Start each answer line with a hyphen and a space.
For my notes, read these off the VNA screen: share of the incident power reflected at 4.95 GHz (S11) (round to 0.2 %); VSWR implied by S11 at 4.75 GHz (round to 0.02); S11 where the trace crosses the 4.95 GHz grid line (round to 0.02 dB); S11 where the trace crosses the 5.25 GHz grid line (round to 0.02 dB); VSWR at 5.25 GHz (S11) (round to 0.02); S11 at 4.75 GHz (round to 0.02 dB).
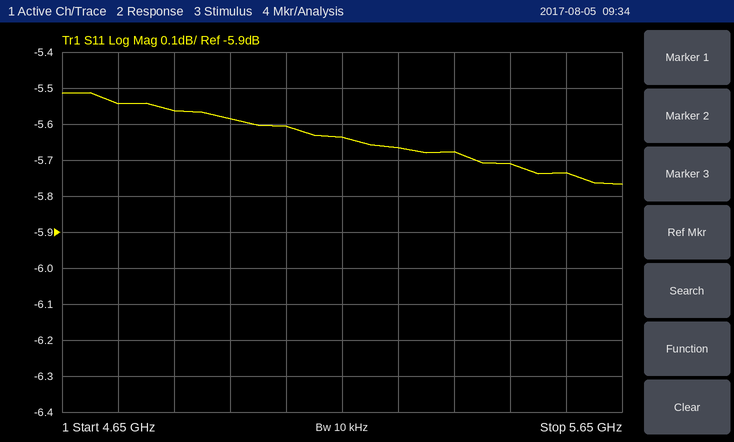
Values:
- 27.6 %
- 3.24
- -5.58 dB
- -5.66 dB
- 3.18
- -5.54 dB
